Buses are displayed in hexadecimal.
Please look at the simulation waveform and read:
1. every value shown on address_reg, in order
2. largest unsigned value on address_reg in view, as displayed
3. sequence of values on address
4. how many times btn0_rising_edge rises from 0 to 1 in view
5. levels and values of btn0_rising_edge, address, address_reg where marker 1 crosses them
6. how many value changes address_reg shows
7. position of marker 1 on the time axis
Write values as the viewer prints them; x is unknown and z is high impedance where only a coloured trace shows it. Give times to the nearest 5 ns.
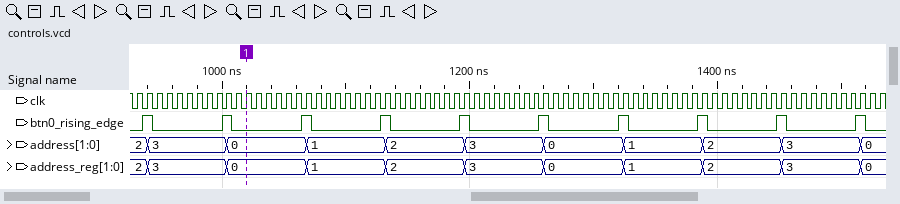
2, 3, 0, 1, 2, 3, 0, 1, 2, 3, 0
3
2, 3, 0, 1, 2, 3, 0, 1, 2, 3, 0
10
btn0_rising_edge=0, address=0, address_reg=0
10
1020 ns
